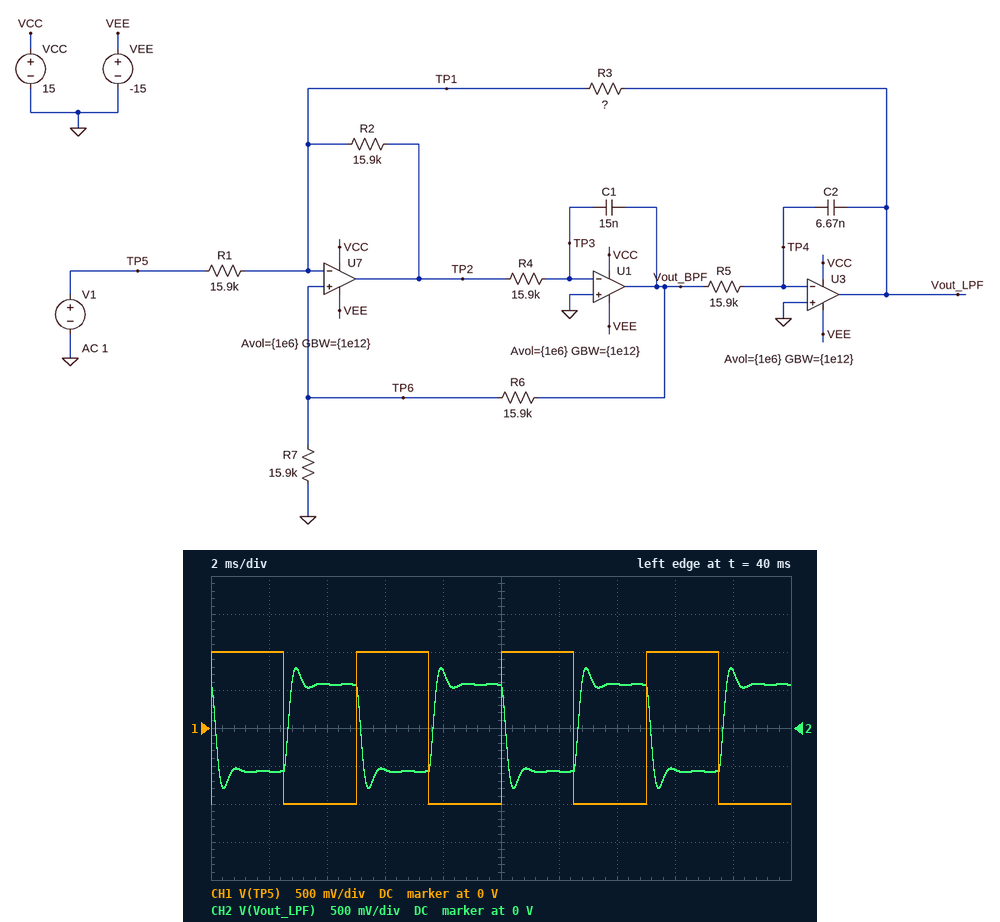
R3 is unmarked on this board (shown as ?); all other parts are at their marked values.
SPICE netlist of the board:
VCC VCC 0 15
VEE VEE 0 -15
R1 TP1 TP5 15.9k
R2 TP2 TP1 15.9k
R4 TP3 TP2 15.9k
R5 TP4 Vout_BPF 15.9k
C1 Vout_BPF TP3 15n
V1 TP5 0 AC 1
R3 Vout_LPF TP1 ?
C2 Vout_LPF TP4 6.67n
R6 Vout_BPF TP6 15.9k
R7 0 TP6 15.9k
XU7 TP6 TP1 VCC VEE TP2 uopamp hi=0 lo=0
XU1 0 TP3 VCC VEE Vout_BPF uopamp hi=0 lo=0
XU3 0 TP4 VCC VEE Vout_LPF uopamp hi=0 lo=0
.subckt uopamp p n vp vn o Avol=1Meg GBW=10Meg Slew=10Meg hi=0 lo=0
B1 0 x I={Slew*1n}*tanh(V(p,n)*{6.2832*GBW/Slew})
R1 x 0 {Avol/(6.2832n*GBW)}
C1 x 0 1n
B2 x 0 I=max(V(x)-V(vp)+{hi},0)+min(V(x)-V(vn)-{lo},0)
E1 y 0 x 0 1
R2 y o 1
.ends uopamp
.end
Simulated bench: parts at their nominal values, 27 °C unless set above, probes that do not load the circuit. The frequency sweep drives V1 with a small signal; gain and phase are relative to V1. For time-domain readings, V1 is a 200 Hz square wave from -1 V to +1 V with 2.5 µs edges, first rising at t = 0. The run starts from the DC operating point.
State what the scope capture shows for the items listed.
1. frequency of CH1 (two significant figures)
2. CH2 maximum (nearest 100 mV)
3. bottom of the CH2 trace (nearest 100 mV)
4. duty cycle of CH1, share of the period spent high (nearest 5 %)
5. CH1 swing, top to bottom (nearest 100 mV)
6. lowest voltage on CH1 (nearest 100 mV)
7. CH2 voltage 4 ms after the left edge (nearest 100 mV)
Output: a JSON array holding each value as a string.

["200 Hz", "800 mV", "-800 mV", "50 %", "2.0 V", "-1.0 V", "600 mV"]
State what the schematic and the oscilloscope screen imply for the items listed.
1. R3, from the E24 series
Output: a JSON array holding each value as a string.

["9.1 kΩ"]
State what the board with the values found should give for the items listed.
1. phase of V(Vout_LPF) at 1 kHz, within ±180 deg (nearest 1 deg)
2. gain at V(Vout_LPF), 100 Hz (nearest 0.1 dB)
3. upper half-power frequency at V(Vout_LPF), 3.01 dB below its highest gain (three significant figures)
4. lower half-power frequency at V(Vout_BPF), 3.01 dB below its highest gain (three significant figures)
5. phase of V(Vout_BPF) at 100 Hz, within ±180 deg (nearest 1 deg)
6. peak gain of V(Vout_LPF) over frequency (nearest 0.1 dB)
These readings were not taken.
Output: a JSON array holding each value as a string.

["121 deg", "-4.8 dB", "1.56 kHz", "838 Hz", "86 deg", "-3.3 dB"]
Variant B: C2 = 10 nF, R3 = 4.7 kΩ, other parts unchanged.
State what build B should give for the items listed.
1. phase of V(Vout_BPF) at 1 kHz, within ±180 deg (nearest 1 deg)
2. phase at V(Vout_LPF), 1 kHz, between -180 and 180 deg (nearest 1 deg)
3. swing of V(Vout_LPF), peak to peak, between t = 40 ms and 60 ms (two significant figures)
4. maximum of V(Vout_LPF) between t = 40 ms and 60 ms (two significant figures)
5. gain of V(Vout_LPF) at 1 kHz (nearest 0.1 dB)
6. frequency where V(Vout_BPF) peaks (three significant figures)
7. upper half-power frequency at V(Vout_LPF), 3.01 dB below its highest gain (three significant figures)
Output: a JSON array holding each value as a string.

["35 deg", "125 deg", "710 mV", "350 mV", "-10.3 dB", "1.50 kHz", "1.68 kHz"]
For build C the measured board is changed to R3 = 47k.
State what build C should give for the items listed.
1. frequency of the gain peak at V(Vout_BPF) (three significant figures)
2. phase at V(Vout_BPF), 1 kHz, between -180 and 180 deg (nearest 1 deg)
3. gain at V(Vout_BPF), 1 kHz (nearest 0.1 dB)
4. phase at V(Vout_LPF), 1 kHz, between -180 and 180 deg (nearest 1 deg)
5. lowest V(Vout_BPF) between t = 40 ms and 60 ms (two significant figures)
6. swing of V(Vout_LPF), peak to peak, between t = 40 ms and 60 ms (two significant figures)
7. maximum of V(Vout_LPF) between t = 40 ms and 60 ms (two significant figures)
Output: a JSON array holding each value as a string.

["582 Hz", "-40 deg", "-3.7 dB", "50 deg", "-1.1 V", "6.6 V", "3.3 V"]
